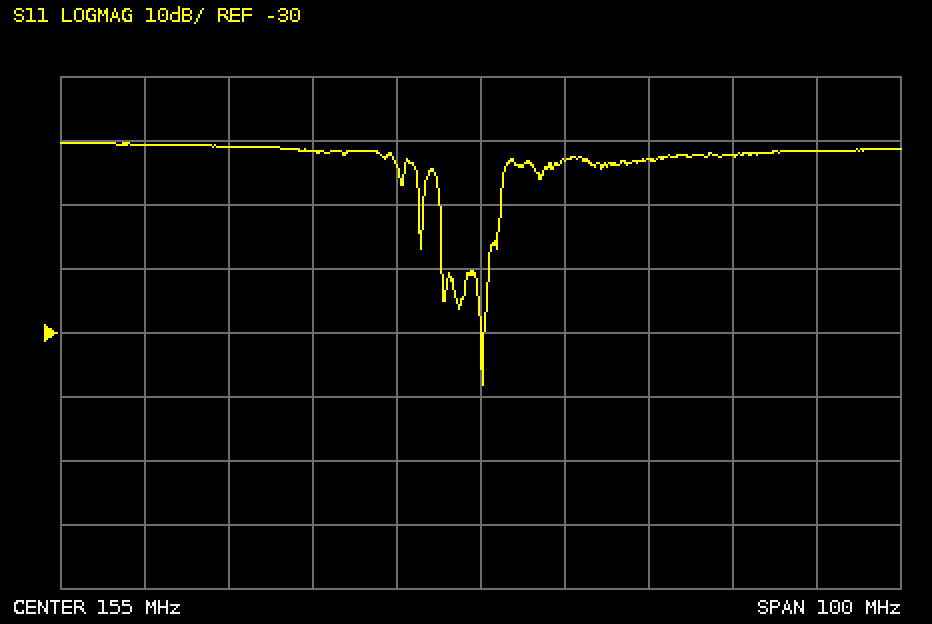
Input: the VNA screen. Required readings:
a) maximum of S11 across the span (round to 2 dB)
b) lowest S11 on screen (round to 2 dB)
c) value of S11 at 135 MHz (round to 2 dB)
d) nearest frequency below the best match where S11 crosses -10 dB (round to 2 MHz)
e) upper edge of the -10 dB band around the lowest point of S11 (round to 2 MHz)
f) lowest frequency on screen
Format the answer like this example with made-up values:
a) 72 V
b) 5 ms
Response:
a) 0 dB
b) -38 dB
c) -2 dB
d) 150 MHz
e) 158 MHz
f) 105 MHz
